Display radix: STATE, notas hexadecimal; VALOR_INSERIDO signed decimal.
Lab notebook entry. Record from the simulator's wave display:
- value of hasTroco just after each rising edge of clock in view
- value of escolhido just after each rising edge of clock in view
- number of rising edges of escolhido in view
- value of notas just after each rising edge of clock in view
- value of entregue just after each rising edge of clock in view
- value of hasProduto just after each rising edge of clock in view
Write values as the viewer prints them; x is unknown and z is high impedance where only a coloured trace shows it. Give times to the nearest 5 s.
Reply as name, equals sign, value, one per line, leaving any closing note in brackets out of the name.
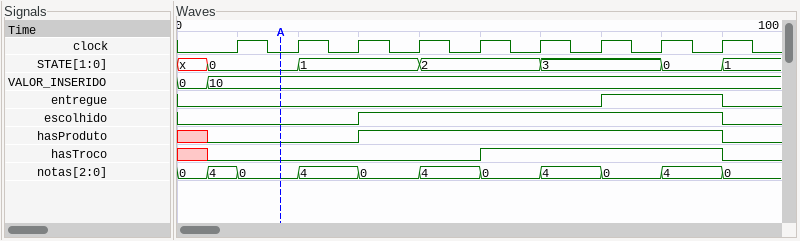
value of hasTroco just after each rising edge of clock in view = 0 0 0 0 1 1 1 1 0
value of escolhido just after each rising edge of clock in view = 0 0 1 1 1 1 1 1 0
number of rising edges of escolhido in view = 1
value of notas just after each rising edge of clock in view = 0, 4, 0, 4, 0, 4, 0, 4, 0
value of entregue just after each rising edge of clock in view = 0 0 0 0 0 0 1 1 0
value of hasProduto just after each rising edge of clock in view = 0 0 1 1 1 1 1 1 0
